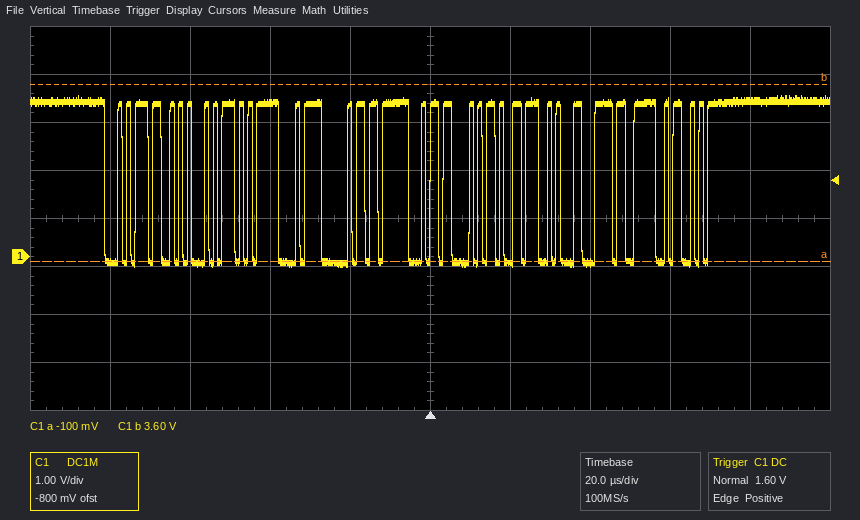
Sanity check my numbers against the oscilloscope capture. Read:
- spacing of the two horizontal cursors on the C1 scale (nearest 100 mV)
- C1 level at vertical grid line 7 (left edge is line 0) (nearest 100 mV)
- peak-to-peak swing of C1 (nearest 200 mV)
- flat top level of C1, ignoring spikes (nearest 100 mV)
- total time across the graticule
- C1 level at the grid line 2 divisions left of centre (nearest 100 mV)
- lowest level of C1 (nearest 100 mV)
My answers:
3.7 V
-100 mV
3.6 V
3.2 V
200 µs
3.2 V
-200 mV
